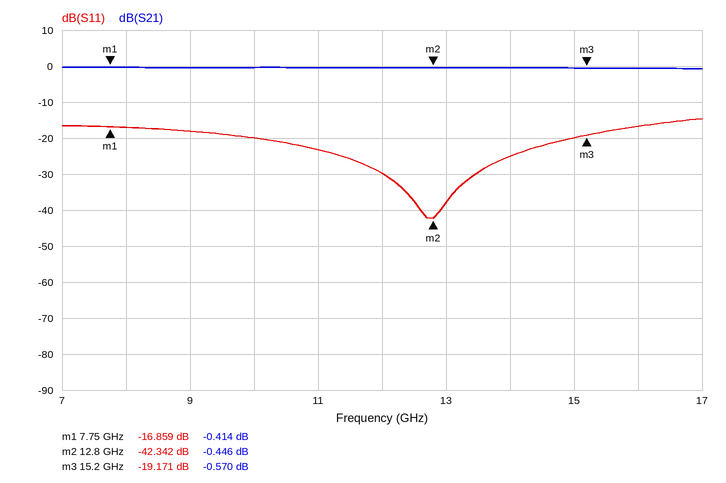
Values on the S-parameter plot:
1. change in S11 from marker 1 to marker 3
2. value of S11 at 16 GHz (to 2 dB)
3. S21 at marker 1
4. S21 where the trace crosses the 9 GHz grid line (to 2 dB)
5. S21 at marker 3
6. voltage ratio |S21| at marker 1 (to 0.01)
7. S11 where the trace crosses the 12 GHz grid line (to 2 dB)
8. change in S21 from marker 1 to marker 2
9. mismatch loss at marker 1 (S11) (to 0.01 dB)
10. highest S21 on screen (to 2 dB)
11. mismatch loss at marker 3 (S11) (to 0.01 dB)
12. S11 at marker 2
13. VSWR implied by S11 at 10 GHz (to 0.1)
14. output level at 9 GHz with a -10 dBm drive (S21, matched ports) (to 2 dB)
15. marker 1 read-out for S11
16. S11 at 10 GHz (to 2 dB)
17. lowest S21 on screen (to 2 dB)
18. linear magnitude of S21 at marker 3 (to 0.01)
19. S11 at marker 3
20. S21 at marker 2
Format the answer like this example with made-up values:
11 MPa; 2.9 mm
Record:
-2.312 dB; -16 dB; -0.414 dB; 0 dB; -0.570 dB; 0.95; -30 dB; -0.032 dB; 0.09 dB; 0 dB; 0.05 dB; -42.342 dB; 1.2; -10 dBm; -16.859 dB; -20 dB; 0 dB; 0.94; -19.171 dB; -0.446 dB
